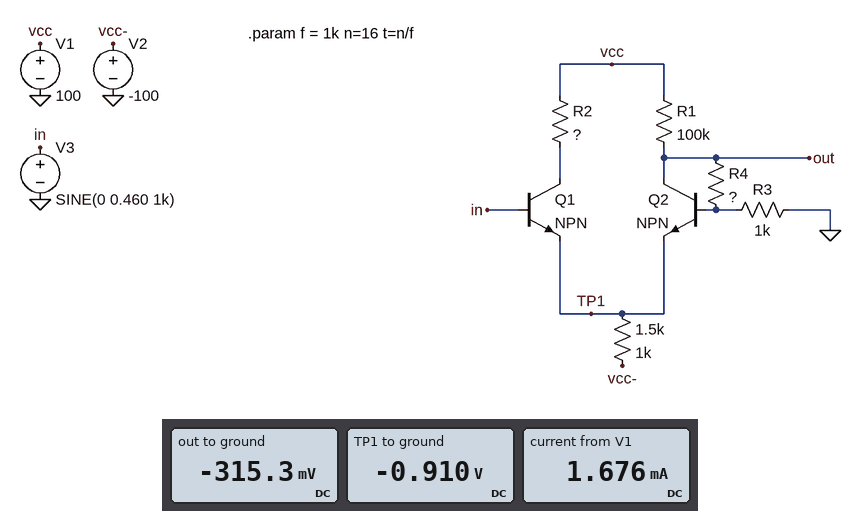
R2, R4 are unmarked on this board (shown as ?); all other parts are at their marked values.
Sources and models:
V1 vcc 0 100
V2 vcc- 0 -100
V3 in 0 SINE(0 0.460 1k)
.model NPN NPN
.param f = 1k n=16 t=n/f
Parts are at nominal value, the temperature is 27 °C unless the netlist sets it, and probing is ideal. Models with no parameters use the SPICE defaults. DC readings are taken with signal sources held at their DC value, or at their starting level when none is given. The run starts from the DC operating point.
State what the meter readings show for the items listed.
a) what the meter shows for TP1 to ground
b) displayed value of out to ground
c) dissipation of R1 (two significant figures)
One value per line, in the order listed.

-0.910 V
-315.3 mV
100 mW
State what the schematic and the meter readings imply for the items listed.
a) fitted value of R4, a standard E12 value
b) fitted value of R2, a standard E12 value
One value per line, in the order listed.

1.5 kΩ
150 kΩ
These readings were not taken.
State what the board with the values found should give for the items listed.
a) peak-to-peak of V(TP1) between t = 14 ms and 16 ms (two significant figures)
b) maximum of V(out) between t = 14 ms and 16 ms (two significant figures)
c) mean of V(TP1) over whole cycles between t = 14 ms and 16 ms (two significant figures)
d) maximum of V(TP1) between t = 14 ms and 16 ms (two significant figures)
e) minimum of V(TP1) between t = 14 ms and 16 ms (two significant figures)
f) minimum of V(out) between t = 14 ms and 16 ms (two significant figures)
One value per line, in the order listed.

920 mV
790 mV
-910 mV
-450 mV
-1.4 V
-1.3 V
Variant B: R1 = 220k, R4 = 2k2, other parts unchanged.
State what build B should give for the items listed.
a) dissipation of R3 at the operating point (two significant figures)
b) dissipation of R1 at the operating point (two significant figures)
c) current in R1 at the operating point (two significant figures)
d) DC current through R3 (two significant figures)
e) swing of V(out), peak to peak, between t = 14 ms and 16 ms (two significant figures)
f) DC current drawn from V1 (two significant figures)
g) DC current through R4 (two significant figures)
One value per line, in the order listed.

22 µW
46 mW
460 µA
150 µA
2.2 V
1.1 mA
140 µA
